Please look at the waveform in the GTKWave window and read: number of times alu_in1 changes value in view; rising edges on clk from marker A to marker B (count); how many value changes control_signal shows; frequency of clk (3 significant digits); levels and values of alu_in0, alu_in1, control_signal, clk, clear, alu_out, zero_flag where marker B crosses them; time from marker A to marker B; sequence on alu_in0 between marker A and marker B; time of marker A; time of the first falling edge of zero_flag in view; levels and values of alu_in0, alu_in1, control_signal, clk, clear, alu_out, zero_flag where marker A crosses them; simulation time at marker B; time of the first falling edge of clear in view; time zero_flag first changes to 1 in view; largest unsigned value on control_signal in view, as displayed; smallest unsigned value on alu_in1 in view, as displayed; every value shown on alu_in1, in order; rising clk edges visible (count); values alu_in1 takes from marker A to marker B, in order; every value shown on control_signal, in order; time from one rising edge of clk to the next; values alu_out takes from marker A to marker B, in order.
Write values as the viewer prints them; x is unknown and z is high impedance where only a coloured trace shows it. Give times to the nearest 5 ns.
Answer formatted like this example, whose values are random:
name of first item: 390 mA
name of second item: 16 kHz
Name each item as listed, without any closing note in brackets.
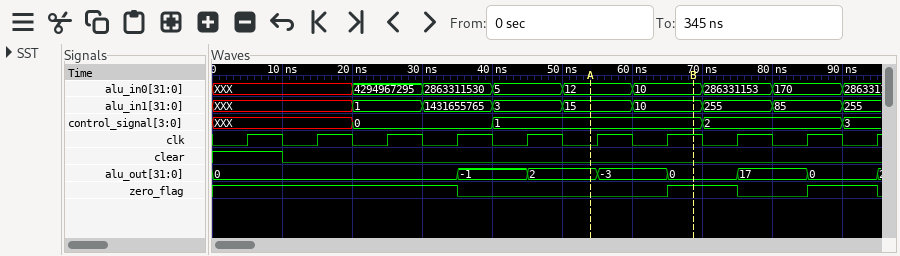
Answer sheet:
number of times alu_in1 changes value in view: 8
rising edges on clk from marker A to marker B: 2
how many value changes control_signal shows: 4
frequency of clk: 100 MHz
levels and values of alu_in0, alu_in1, control_signal, clk, clear, alu_out, zero_flag where marker B crosses them: alu_in0=10, alu_in1=10, control_signal=1, clk=1, clear=0, alu_out=0, zero_flag=1
time from marker A to marker B: 15 ns
sequence on alu_in0 between marker A and marker B: 12, 10
time of marker A: 55 ns
time of the first falling edge of zero_flag in view: 35 ns
levels and values of alu_in0, alu_in1, control_signal, clk, clear, alu_out, zero_flag where marker A crosses them: alu_in0=12, alu_in1=15, control_signal=1, clk=0, clear=0, alu_out=2, zero_flag=0
simulation time at marker B: 70 ns
time of the first falling edge of clear in view: 10 ns
time zero_flag first changes to 1 in view: 65 ns
largest unsigned value on control_signal in view, as displayed: 3
smallest unsigned value on alu_in1 in view, as displayed: 1
every value shown on alu_in1, in order: XXX, 1, 1431655765, 3, 15, 10, 255, 85, 255
rising clk edges visible: 10
values alu_in1 takes from marker A to marker B, in order: 15, 10
every value shown on control_signal, in order: XXX, 0, 1, 2, 3
time from one rising edge of clk to the next: 10 ns
values alu_out takes from marker A to marker B, in order: 2, -3, 0
